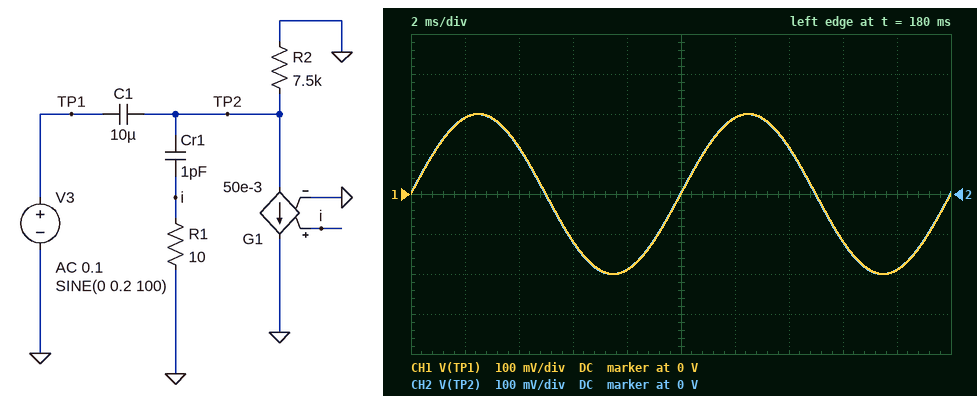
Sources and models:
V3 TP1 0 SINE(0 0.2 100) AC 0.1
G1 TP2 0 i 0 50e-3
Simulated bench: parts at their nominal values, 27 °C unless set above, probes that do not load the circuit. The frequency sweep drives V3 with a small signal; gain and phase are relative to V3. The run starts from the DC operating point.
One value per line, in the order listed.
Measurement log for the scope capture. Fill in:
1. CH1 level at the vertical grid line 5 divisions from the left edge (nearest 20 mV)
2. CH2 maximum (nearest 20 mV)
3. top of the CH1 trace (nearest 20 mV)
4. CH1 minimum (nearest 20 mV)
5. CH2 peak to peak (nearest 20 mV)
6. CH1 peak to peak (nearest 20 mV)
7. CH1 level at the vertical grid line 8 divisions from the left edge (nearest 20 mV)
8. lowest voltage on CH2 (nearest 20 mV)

0 V
200 mV
200 mV
-200 mV
400 mV
400 mV
-120 mV
-200 mV
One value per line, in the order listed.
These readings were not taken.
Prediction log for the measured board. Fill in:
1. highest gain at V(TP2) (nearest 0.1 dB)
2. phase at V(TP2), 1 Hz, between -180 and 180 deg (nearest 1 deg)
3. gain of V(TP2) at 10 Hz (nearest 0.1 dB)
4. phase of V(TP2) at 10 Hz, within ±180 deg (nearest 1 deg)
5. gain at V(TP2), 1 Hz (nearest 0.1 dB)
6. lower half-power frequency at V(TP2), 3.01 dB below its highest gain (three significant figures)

0 dB
65 deg
-0.2 dB
12 deg
-7.4 dB
2.12 Hz
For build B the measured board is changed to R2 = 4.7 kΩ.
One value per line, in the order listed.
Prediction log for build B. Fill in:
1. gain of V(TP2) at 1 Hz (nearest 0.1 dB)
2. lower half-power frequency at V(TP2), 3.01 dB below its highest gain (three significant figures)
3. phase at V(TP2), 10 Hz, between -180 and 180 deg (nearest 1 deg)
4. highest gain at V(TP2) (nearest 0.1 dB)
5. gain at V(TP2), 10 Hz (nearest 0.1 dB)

-11.0 dB
3.39 Hz
19 deg
0 dB
-0.5 dB
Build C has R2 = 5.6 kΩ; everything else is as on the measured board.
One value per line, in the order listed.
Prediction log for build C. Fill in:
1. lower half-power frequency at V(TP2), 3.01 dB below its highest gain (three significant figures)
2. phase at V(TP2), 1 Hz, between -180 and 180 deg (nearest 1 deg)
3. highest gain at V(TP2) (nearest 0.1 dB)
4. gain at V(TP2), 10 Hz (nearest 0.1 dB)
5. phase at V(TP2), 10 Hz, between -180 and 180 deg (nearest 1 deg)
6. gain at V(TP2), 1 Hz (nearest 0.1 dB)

2.84 Hz
71 deg
0 dB
-0.3 dB
16 deg
-9.6 dB
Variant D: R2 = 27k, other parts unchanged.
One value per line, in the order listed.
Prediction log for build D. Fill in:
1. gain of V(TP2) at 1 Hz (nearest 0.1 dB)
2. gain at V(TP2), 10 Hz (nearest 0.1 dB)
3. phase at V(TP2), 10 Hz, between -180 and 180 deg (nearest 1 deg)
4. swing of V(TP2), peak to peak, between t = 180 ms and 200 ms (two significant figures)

-1.3 dB
0 dB
3 deg
400 mV
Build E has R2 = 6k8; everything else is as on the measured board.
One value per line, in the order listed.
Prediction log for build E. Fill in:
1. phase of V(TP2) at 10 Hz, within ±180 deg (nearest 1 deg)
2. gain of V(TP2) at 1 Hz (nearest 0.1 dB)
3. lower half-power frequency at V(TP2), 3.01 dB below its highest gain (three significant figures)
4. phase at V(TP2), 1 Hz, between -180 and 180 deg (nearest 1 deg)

13 deg
-8.1 dB
2.34 Hz
67 deg
